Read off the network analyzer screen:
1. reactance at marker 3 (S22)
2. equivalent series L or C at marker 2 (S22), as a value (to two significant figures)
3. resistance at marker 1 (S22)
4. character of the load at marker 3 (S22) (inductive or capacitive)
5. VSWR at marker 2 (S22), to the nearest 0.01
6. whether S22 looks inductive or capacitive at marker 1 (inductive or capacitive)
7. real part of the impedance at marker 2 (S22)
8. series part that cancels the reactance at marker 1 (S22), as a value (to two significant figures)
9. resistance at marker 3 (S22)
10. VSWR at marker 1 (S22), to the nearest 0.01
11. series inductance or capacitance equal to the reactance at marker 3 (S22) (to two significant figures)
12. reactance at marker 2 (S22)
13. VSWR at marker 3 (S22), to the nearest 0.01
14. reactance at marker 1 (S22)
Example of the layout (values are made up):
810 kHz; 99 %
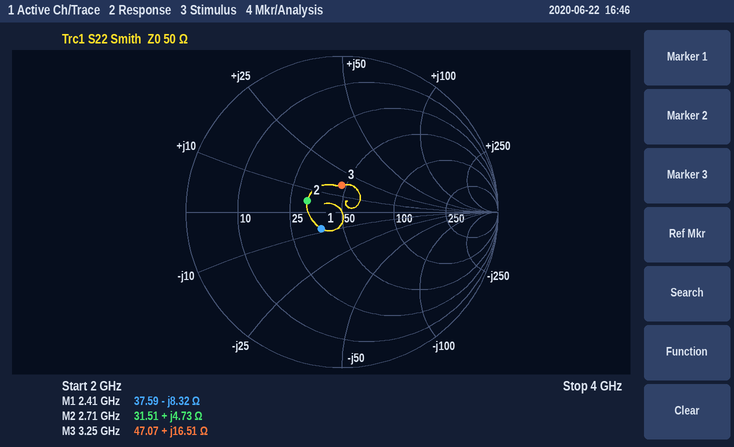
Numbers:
+16.51 Ω; 280 pH; 37.59 Ω; inductive; 1.61; capacitive; 31.51 Ω; 550 pH; 47.07 Ω; 1.41; 810 pH; +4.73 Ω; 1.41; -8.32 Ω
